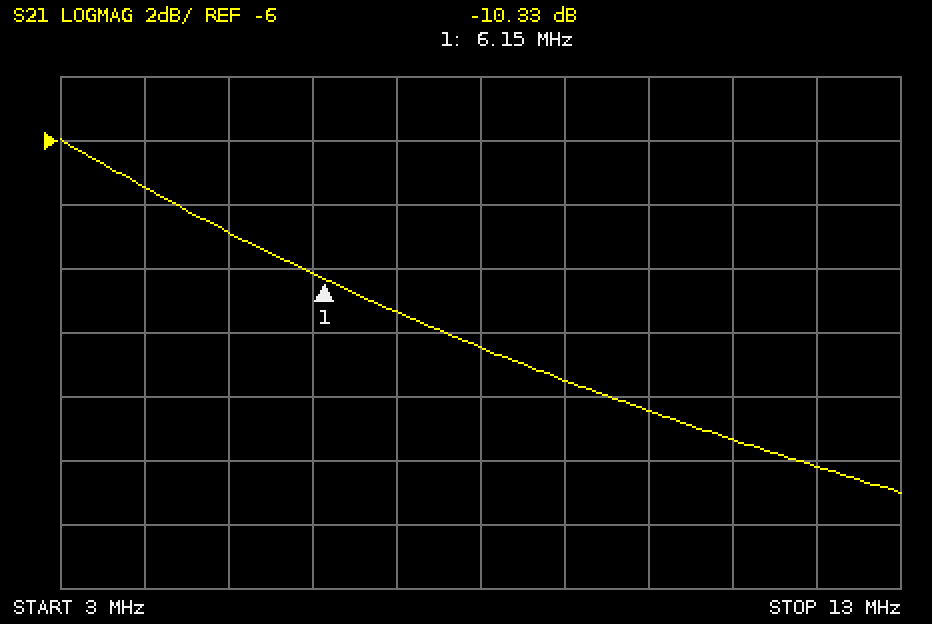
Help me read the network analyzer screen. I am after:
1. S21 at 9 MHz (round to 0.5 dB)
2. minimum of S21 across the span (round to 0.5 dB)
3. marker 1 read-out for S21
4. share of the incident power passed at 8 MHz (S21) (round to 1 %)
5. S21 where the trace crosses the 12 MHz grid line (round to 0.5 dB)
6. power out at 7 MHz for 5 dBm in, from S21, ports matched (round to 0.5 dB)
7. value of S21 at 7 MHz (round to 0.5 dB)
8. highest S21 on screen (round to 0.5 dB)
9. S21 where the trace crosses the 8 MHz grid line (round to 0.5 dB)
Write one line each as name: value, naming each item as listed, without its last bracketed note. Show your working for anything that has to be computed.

S21 at 9 MHz: -13.5 dB
minimum of S21 across the span: -17.0 dB
marker 1 read-out for S21: -10.33 dB
share of the incident power passed at 8 MHz (S21): 10^(-12.5/10) ≈ 6 %
S21 where the trace crosses the 12 MHz grid line: -16.0 dB
power out at 7 MHz for 5 dBm in, from S21, ports matched: 5 dBm + (-11.5 dB) = -6.5 dBm
value of S21 at 7 MHz: -11.5 dB
highest S21 on screen: -6.0 dB
S21 where the trace crosses the 8 MHz grid line: -12.5 dB
